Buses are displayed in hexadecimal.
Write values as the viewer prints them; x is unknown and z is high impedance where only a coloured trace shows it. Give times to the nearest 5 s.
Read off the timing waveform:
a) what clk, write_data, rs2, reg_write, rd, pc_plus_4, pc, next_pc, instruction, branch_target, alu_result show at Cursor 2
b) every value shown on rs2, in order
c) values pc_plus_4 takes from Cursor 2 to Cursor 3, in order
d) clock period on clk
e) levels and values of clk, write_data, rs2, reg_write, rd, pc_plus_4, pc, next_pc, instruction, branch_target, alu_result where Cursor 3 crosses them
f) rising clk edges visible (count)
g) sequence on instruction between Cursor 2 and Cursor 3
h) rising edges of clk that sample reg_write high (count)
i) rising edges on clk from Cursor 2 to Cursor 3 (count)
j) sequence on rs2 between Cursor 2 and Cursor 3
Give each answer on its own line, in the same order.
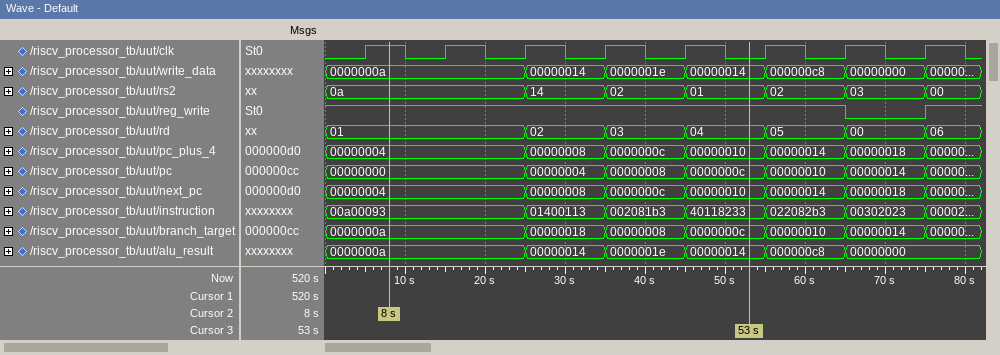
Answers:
clk=1, write_data=0000000a, rs2=0a, reg_write=1, rd=01, pc_plus_4=00000004, pc=00000000, next_pc=00000004, instruction=00a00093, branch_target=0000000a, alu_result=0000000a
0a, 14, 02, 01, 02, 03, 00
00000004, 00000008, 0000000c, 00000010
10 s
clk=0, write_data=00000014, rs2=01, reg_write=1, rd=04, pc_plus_4=00000010, pc=0000000c, next_pc=00000010, instruction=40118233, branch_target=0000000c, alu_result=00000014
8
00a00093, 01400113, 002081b3, 40118233
7
4
0a, 14, 02, 01
